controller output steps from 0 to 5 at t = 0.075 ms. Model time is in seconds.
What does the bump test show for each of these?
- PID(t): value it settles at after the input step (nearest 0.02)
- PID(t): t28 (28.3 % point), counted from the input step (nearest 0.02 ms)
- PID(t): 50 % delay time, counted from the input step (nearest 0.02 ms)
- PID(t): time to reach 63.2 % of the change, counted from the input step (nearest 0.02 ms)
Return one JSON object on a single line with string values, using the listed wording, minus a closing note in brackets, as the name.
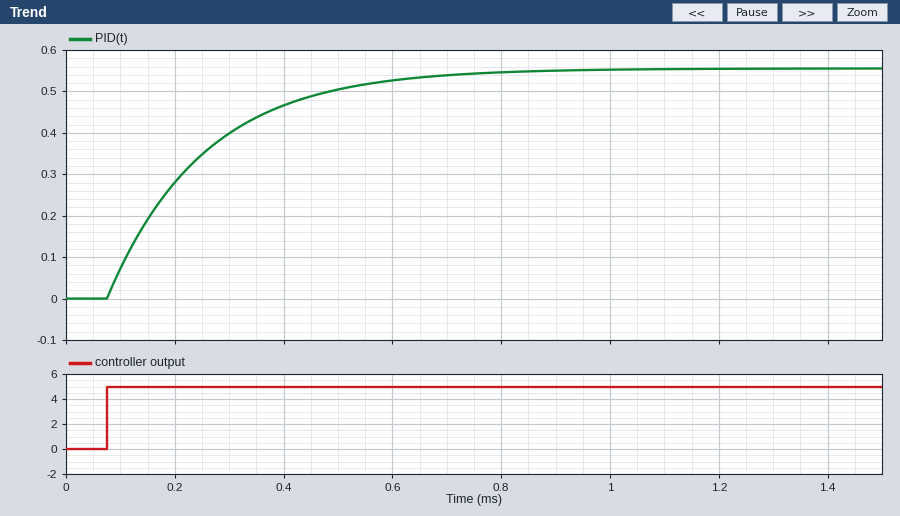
{"PID(t): value it settles at after the input step": "0.56", "PID(t): t28 (28.3 % point), counted from the input step": "0.06 ms", "PID(t): 50 % delay time, counted from the input step": "0.12 ms", "PID(t): time to reach 63.2 % of the change, counted from the input step": "0.18 ms"}
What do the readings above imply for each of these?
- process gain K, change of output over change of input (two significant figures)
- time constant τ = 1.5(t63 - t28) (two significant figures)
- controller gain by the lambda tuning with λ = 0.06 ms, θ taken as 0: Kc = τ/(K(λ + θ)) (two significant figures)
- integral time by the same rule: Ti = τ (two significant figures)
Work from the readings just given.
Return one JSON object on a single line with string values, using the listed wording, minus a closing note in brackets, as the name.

{"process gain K, change of output over change of input": "0.11", "time constant τ = 1.5(t63 - t28)": "0.18 ms", "controller gain by the lambda tuning with λ = 0.06 ms, θ taken as 0: Kc = τ/(K(λ + θ))": "27", "integral time by the same rule: Ti = τ": "0.18 ms"}
